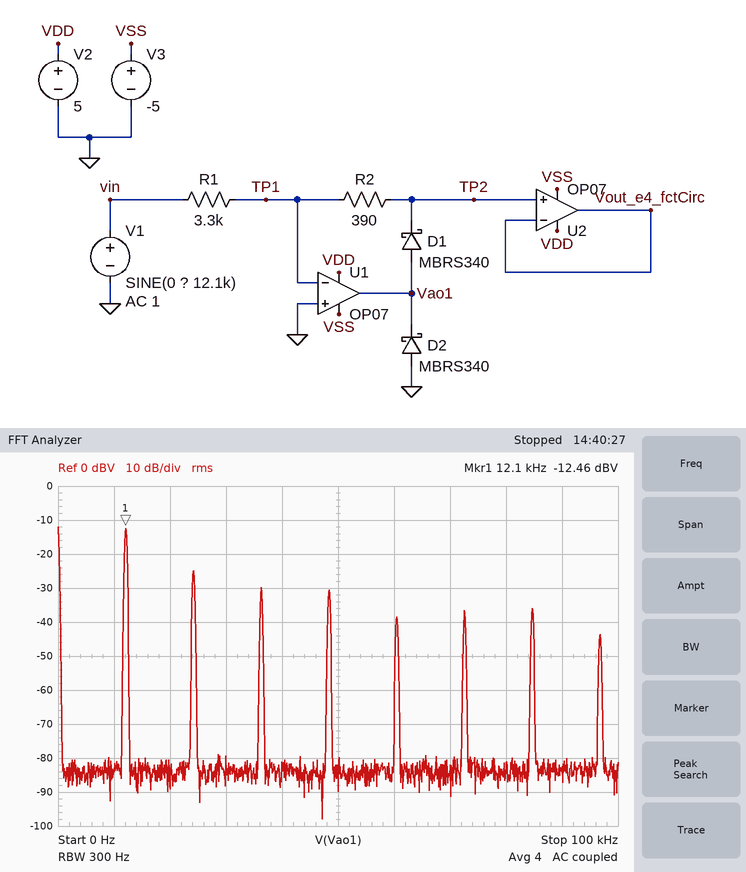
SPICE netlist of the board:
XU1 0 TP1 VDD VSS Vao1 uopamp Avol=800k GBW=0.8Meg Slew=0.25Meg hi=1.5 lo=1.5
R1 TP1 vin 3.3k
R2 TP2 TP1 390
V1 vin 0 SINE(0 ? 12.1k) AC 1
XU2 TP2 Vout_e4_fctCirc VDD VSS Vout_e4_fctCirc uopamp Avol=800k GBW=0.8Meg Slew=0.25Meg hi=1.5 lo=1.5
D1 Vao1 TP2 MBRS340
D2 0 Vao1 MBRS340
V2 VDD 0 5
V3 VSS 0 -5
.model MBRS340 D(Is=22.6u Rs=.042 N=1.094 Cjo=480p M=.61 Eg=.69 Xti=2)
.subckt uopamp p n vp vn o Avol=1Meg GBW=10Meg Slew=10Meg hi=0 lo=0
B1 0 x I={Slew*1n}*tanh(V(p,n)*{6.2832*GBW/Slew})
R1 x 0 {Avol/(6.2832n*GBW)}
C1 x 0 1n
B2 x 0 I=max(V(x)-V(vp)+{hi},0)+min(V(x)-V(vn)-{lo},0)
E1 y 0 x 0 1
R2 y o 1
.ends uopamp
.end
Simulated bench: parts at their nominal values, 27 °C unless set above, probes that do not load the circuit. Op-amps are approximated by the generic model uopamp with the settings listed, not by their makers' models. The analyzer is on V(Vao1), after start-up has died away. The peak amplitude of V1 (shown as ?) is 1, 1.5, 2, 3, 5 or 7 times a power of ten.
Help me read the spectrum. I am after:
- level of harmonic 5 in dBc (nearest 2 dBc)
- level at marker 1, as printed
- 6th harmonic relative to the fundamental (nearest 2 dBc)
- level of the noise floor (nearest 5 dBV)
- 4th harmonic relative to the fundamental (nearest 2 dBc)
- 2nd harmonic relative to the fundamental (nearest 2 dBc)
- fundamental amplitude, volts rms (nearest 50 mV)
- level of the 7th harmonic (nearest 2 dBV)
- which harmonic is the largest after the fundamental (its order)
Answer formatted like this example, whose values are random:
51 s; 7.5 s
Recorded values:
-26 dBc; -12.46 dBV; -24 dBc; -85 dBV; -18 dBc; -12 dBc; 250 mV; -36 dBV; 2
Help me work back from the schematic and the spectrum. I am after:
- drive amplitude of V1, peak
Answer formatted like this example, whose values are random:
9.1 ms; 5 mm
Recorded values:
700 mV
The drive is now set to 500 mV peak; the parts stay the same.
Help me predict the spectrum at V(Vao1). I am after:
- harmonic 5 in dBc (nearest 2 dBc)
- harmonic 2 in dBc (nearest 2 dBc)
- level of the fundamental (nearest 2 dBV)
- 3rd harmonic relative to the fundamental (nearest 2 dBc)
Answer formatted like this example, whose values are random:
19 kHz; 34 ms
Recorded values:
-28 dBc; -14 dBc; -12 dBV; -16 dBc
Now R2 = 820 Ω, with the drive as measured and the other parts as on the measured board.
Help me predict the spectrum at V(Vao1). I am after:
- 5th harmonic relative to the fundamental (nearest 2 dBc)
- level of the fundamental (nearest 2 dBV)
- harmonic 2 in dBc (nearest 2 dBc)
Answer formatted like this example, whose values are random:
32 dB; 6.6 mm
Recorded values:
-24 dBc; -12 dBV; -10 dBc
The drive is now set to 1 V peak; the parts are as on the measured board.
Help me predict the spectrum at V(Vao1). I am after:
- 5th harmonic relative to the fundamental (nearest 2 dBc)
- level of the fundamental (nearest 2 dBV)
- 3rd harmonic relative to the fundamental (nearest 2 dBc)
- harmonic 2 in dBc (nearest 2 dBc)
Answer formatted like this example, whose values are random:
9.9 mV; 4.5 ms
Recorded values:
-24 dBc; -12 dBV; -18 dBc; -10 dBc
